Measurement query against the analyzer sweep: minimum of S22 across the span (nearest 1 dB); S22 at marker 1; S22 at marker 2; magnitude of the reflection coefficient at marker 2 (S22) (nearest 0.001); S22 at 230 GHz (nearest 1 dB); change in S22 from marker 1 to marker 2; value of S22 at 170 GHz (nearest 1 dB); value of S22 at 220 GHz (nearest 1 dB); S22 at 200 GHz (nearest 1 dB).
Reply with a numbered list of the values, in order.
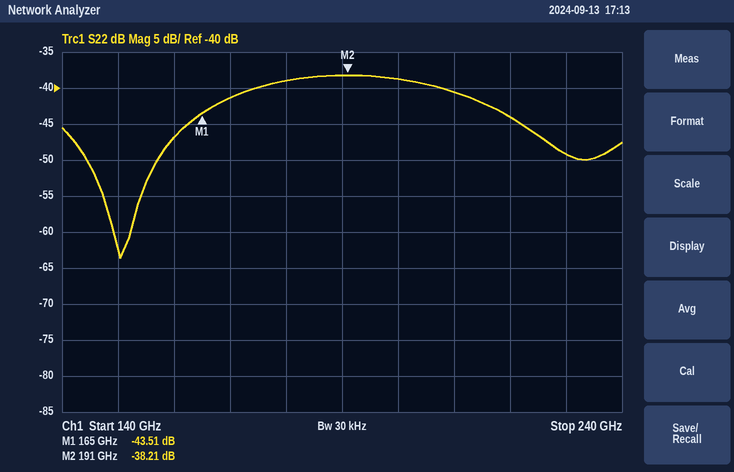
1. -64 dB
2. -43.51 dB
3. -38.21 dB
4. 0.012
5. -49 dB
6. 5.30 dB
7. -41 dB
8. -44 dB
9. -39 dB
